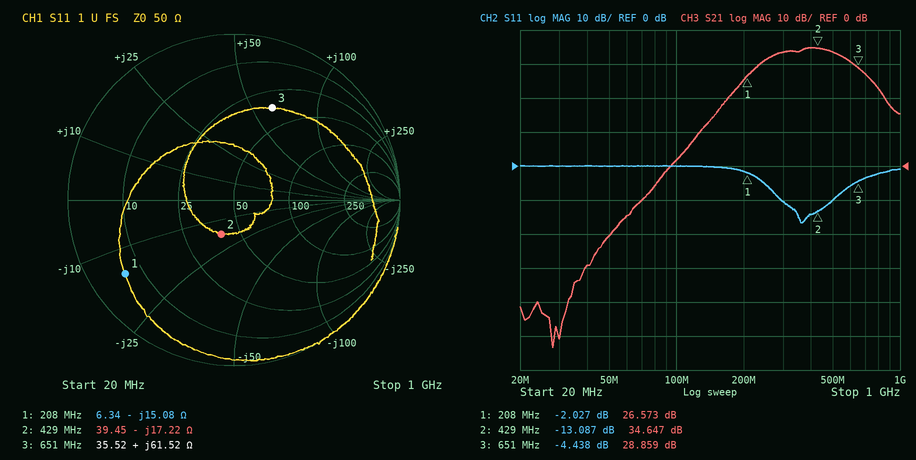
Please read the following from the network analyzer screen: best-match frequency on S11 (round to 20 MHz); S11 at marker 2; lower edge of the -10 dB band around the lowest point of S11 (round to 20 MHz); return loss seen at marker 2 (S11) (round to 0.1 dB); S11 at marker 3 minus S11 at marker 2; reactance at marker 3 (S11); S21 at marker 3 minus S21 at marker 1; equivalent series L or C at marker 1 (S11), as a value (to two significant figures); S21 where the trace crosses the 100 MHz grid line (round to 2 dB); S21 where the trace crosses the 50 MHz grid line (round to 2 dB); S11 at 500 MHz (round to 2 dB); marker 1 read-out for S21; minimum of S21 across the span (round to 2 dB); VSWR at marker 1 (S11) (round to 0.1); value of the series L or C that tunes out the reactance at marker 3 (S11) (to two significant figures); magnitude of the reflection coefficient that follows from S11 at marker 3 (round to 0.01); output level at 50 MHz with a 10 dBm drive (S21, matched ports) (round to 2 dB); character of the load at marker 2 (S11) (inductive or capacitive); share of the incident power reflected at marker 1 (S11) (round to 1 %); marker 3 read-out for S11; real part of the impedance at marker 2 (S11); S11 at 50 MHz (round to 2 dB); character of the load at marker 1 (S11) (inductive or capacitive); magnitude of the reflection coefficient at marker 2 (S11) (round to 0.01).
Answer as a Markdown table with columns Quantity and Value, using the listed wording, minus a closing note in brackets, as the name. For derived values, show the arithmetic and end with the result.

| Quantity | Value |
|---|---|
| best-match frequency on S11 | 360 MHz |
| S11 at marker 2 | -13.087 dB |
| lower edge of the -10 dB band around the lowest point of S11 | 300 MHz |
| return loss seen at marker 2 (S11) | 13.1 dB |
| S11 at marker 3 minus S11 at marker 2 | -4.438 − (-13.087) = 8.649 dB |
| reactance at marker 3 | +61.52 Ω |
| S21 at marker 3 minus S21 at marker 1 | 28.859 − (26.573) = 2.286 dB |
| equivalent series L or C at marker 1 (S11), as a value | C = 1/(2π × 208 MHz × 15.08 Ω) ≈ 51 pF |
| S21 where the trace crosses the 100 MHz grid line | 2 dB |
| S21 where the trace crosses the 50 MHz grid line | -20 dB |
| S11 at 500 MHz | -10 dB |
| marker 1 read-out for S21 | 26.573 dB |
| minimum of S21 across the span | -54 dB |
| VSWR at marker 1 (S11) | 8.6 |
| value of the series L or C that tunes out the reactance at marker 3 (S11) | C = 1/(2π × 651 MHz × 61.52 Ω) ≈ 4.0 pF |
| magnitude of the reflection coefficient that follows from S11 at marker 3 | 10^(-4.438/20) ≈ 0.60 |
| output level at 50 MHz with a 10 dBm drive (S21, matched ports) | 10 dBm + (-20 dB) = -10 dBm |
| character of the load at marker 2 (S11) | capacitive |
| share of the incident power reflected at marker 1 (S11) | 10^(-2.027/10) ≈ 63 % |
| marker 3 read-out for S11 | -4.438 dB |
| real part of the impedance at marker 2 | 39.45 Ω |
| S11 at 50 MHz | 0 dB |
| character of the load at marker 1 (S11) | capacitive |
| magnitude of the reflection coefficient at marker 2 (S11) | 10^(-13.087/20) ≈ 0.22 |
